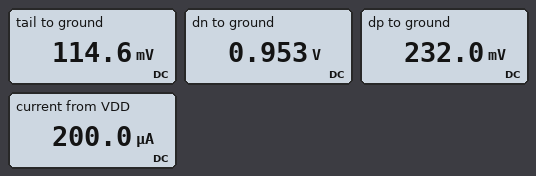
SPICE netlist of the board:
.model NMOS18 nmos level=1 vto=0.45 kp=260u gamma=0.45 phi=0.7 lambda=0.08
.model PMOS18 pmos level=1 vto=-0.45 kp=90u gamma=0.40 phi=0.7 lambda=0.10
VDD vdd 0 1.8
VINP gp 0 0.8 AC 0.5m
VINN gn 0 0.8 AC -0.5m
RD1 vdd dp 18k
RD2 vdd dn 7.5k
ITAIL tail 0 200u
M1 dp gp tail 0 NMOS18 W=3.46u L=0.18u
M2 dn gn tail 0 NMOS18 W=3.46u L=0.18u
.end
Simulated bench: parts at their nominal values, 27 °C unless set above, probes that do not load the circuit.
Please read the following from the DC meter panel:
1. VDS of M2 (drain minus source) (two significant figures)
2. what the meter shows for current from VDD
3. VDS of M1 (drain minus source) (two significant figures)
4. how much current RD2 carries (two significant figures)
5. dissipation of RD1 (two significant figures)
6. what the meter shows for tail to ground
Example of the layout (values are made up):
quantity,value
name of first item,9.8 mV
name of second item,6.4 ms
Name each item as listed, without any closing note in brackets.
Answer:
quantity,value
VDS of M2 (drain minus source),840 mV
what the meter shows for current from VDD,200.0 µA
VDS of M1 (drain minus source),120 mV
how much current RD2 carries,110 µA
dissipation of RD1,140 µW
what the meter shows for tail to ground,114.6 mV
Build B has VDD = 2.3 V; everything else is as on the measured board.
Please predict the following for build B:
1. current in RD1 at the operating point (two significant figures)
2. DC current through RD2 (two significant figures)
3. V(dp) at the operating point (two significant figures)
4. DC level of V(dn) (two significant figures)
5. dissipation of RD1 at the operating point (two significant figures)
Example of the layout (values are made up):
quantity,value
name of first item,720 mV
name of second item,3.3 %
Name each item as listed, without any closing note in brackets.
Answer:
quantity,value
current in RD1 at the operating point,96 µA
DC current through RD2,100 µA
V(dp) at the operating point,560 mV
DC level of V(dn),1.5 V
dissipation of RD1 at the operating point,170 µW
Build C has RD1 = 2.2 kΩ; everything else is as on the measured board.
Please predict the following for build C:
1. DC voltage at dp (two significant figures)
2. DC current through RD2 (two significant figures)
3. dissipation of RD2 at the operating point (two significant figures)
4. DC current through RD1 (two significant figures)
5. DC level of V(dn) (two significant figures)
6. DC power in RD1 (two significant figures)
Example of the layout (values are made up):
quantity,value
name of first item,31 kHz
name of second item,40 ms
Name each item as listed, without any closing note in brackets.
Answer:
quantity,value
DC voltage at dp,1.6 V
DC current through RD2,98 µA
dissipation of RD2 at the operating point,72 µW
DC current through RD1,100 µA
DC level of V(dn),1.1 V
DC power in RD1,23 µW
